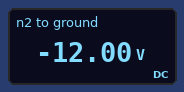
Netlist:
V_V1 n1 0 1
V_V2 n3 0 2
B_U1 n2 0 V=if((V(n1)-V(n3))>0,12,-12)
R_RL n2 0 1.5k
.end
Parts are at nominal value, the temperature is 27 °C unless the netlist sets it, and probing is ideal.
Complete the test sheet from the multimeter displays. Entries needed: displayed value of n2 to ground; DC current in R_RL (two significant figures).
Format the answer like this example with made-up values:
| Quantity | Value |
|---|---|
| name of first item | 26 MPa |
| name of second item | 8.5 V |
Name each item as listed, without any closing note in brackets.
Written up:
| Quantity | Value |
|---|---|
| displayed value of n2 to ground | -12.00 V |
| DC current in R_RL | 8.0 mA |
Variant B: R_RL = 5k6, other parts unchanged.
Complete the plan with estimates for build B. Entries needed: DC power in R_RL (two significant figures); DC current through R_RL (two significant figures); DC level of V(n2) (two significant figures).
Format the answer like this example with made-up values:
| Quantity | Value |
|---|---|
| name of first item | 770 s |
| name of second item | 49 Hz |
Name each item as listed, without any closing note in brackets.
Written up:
| Quantity | Value |
|---|---|
| DC power in R_RL | 26 mW |
| DC current through R_RL | 2.1 mA |
| DC level of V(n2) | -12 V |
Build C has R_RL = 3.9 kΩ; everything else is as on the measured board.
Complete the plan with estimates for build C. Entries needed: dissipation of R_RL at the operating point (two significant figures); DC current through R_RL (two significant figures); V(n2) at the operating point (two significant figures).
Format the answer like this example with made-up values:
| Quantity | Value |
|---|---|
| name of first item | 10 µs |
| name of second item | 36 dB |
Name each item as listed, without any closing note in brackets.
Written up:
| Quantity | Value |
|---|---|
| dissipation of R_RL at the operating point | 37 mW |
| DC current through R_RL | 3.1 mA |
| V(n2) at the operating point | -12 V |
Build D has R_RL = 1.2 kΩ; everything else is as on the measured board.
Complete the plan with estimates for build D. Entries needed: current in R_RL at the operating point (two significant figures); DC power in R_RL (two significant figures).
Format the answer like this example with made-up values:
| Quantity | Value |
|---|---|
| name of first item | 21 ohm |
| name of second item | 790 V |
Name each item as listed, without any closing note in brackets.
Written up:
| Quantity | Value |
|---|---|
| current in R_RL at the operating point | 10 mA |
| DC power in R_RL | 120 mW |
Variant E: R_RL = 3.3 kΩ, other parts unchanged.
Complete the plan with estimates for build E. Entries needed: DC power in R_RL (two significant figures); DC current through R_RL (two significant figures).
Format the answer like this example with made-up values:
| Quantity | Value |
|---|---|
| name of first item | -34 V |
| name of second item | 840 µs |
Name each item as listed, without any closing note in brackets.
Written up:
| Quantity | Value |
|---|---|
| DC power in R_RL | 44 mW |
| DC current through R_RL | 3.6 mA |
